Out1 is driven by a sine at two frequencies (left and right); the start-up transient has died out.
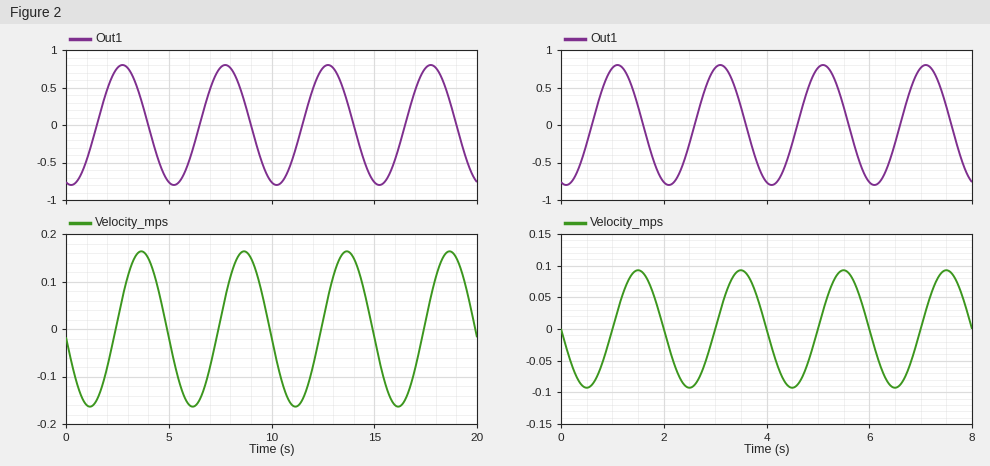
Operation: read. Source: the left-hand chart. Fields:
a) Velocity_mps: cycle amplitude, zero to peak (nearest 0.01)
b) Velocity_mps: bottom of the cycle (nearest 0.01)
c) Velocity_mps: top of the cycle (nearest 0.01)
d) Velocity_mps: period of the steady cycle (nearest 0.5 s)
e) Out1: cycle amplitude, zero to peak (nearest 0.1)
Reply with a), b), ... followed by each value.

a) 0.16
b) -0.16
c) 0.16
d) 5.0 s
e) 0.8
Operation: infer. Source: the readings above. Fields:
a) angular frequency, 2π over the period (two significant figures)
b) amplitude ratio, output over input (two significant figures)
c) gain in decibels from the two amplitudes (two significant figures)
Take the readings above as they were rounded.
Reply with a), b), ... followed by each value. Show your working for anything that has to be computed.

a) 2π / 5 = 1.3 rad/s
b) 0.16 / 0.8 = 0.20
c) 20 log10(0.16 / 0.8) = -14 dB
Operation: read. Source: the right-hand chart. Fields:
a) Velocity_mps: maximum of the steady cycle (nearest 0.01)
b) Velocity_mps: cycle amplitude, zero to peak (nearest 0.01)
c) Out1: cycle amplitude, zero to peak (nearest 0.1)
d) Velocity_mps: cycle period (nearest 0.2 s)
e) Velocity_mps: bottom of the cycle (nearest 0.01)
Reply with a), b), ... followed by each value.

a) 0.09
b) 0.09
c) 0.8
d) 2.0 s
e) -0.09
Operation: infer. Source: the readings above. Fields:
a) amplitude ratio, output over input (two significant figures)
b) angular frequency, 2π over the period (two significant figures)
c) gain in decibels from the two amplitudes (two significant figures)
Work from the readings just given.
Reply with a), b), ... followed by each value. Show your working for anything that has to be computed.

a) 0.09 / 0.8 = 0.11
b) 2π / 2 = 3.1 rad/s
c) 20 log10(0.09 / 0.8) = -19 dB
